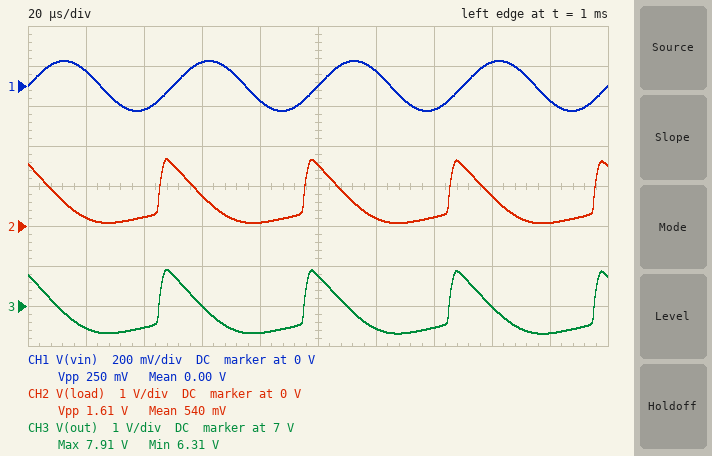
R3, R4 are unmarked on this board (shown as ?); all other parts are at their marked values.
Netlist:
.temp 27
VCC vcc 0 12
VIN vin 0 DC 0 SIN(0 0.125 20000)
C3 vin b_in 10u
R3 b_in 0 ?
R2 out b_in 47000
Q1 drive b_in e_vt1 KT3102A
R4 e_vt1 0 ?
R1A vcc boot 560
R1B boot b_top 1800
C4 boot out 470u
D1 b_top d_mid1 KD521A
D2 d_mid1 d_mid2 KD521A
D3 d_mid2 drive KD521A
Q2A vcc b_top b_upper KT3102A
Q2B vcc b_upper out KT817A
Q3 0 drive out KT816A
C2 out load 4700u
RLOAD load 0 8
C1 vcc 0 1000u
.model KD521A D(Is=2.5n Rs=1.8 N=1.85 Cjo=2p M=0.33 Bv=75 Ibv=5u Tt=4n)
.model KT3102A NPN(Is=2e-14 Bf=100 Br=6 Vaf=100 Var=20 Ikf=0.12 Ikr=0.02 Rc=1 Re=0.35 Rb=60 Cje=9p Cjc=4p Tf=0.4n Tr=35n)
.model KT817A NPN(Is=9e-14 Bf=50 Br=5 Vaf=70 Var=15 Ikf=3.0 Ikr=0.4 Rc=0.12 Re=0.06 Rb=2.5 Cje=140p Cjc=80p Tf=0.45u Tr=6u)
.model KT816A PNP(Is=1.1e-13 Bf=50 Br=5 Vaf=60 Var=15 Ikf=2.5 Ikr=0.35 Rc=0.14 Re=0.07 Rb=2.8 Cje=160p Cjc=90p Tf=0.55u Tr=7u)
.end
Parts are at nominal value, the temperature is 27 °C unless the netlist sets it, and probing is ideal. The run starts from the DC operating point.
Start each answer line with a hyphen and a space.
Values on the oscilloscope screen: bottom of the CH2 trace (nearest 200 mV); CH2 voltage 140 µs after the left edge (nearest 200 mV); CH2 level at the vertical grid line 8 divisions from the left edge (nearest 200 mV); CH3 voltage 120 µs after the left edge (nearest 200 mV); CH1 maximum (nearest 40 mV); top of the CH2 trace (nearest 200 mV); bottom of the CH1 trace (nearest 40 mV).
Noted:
- 0 V
- 200 mV
- 800 mV
- 6.4 V
- 120 mV
- 1.6 V
- -120 mV
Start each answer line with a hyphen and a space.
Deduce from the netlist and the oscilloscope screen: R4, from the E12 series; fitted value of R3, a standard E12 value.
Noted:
- 47 Ω
- 8.2 kΩ
